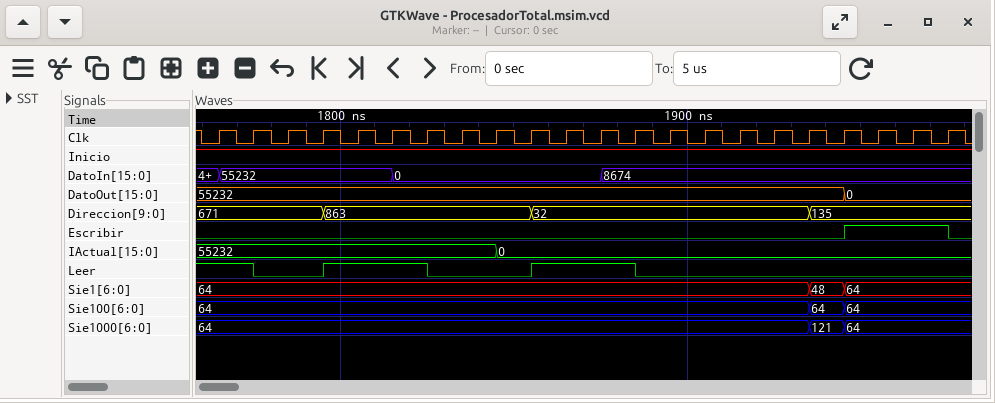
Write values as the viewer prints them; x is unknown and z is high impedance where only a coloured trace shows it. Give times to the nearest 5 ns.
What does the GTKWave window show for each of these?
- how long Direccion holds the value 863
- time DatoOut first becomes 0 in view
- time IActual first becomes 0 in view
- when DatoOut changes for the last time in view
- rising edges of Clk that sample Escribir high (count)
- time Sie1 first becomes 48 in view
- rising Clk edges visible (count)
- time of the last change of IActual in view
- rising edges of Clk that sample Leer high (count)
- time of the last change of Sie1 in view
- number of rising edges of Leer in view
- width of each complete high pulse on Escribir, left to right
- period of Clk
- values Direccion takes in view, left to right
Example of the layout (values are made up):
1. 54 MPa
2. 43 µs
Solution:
1. 60 ns
2. 1945 ns
3. 1845 ns
4. 1945 ns
5. 3
6. 1935 ns
7. 22
8. 1845 ns
9. 8
10. 1945 ns
11. 2
12. 30 ns
13. 10 ns
14. 671, 863, 32, 135
